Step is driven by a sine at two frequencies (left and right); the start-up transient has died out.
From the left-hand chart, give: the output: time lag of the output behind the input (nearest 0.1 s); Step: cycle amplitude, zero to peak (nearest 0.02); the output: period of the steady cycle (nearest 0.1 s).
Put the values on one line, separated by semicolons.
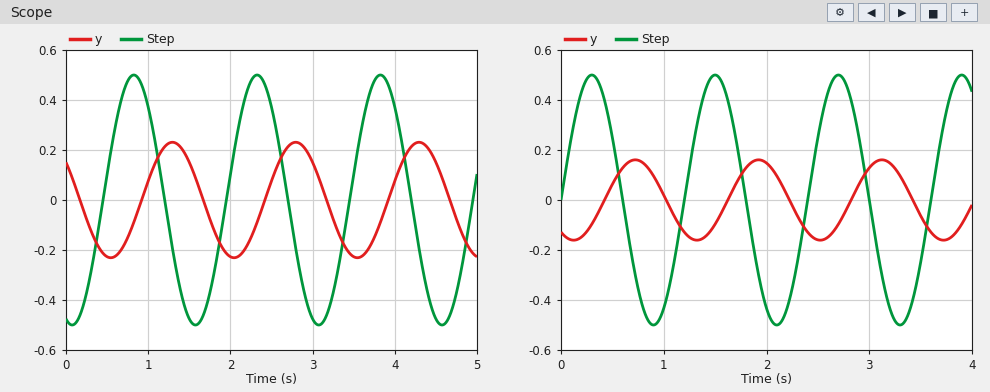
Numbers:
0.5 s; 0.50; 1.5 s
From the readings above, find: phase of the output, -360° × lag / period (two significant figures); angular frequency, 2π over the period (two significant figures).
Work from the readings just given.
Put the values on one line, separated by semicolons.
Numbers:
-120°; 4.2 rad/s
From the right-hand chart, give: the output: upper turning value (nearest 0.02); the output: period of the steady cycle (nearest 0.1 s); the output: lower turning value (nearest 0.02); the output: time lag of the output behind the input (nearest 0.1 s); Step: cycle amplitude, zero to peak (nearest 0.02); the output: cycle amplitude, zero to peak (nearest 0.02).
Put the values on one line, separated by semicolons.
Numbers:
0.16; 1.2 s; -0.16; 0.4 s; 0.50; 0.16
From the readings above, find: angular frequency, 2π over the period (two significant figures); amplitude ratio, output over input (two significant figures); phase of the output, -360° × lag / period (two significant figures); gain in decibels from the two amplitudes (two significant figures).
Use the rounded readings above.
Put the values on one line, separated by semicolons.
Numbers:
5.2 rad/s; 0.32; -120°; -9.9 dB
